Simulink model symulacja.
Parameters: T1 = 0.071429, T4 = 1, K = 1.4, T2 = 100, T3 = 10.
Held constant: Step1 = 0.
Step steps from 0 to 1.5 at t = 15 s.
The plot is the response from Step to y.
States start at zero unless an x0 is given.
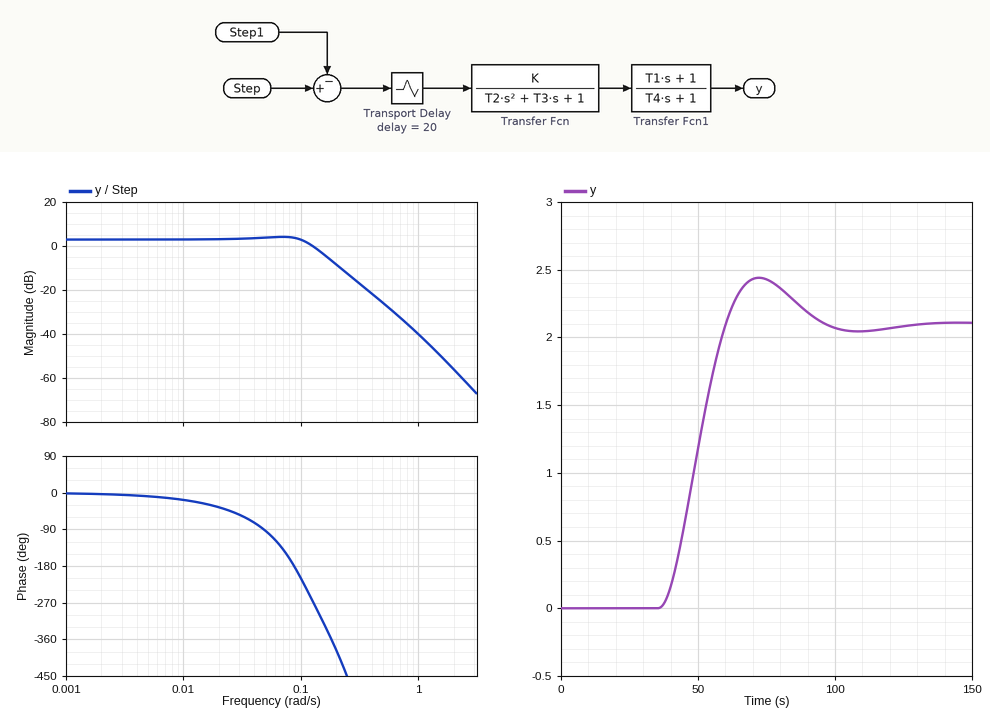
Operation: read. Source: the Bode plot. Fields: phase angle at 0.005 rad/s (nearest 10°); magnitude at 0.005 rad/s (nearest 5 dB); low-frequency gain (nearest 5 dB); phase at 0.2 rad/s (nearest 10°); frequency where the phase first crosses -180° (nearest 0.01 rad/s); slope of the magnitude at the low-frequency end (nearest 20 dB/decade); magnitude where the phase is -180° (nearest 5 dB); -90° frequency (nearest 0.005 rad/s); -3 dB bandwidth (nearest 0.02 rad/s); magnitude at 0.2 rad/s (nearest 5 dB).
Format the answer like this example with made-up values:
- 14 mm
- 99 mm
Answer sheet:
- -10°
- 5 dB
- 5 dB
- -390°
- 0.09 rad/s
- 0 dB/decade
- 5 dB
- 0.050 rad/s
- 0.12 rad/s
- -10 dB
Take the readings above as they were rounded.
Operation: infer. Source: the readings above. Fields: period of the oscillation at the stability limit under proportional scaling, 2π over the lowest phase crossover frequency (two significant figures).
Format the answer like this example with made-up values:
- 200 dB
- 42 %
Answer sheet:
- 70 s
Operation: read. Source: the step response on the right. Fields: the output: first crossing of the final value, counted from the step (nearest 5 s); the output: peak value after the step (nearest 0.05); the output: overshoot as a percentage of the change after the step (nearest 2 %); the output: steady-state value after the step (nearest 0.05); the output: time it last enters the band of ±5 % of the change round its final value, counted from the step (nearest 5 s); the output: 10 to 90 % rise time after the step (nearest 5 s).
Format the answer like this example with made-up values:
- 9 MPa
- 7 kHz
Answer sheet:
- 45 s
- 2.45
- 16 %
- 2.10
- 75 s
- 15 s
